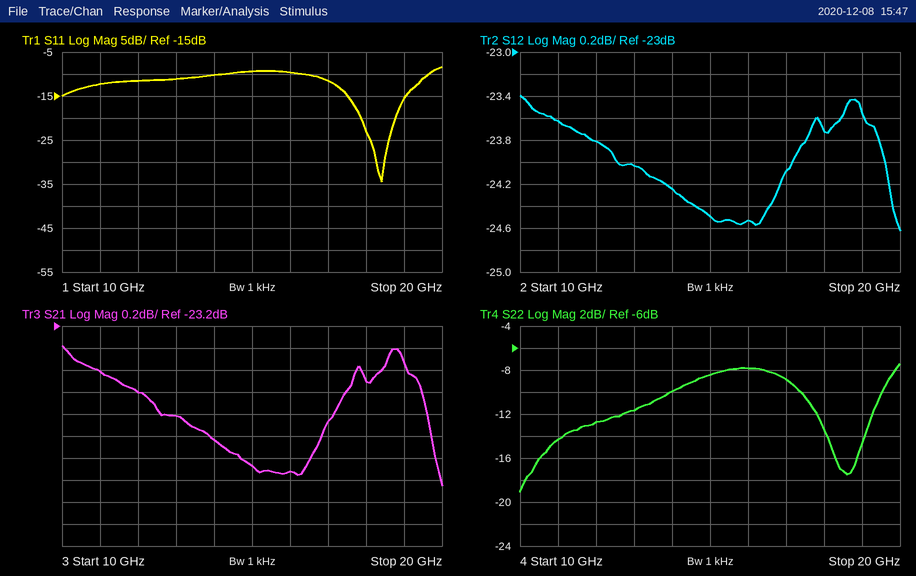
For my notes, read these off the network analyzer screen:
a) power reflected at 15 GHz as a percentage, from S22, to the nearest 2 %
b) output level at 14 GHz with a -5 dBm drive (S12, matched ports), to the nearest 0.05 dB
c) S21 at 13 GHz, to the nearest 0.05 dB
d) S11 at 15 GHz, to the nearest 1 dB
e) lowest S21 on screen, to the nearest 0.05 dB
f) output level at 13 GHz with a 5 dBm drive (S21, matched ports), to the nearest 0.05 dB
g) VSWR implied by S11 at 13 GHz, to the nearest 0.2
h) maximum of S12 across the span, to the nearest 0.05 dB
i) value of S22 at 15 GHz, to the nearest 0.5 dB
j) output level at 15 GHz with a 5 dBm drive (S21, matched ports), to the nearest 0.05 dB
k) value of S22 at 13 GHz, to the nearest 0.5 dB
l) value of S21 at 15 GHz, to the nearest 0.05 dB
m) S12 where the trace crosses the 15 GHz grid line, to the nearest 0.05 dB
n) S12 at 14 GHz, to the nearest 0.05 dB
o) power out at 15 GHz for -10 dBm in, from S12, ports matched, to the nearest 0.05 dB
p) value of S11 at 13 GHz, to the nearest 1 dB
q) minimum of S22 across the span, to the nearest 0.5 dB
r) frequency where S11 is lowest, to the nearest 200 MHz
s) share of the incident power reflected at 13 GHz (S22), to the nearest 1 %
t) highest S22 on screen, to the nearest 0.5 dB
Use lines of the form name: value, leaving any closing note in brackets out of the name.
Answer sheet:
power reflected at 15 GHz as a percentage, from S22, to the nearest 2 %: 14 %
output level at 14 GHz with a -5 dBm drive (S12, matched ports), to the nearest 0.05 dB: -29.25 dBm
S21 at 13 GHz, to the nearest 0.05 dB: -24.00 dB
S11 at 15 GHz, to the nearest 1 dB: -9 dB
lowest S21 on screen, to the nearest 0.05 dB: -24.65 dB
output level at 13 GHz with a 5 dBm drive (S21, matched ports), to the nearest 0.05 dB: -19.00 dBm
VSWR implied by S11 at 13 GHz, to the nearest 0.2: 1.8
maximum of S12 across the span, to the nearest 0.05 dB: -23.40 dB
value of S22 at 15 GHz, to the nearest 0.5 dB: -8.5 dB
output level at 15 GHz with a 5 dBm drive (S21, matched ports), to the nearest 0.05 dB: -19.45 dBm
value of S22 at 13 GHz, to the nearest 0.5 dB: -11.5 dB
value of S21 at 15 GHz, to the nearest 0.05 dB: -24.45 dB
S12 where the trace crosses the 15 GHz grid line, to the nearest 0.05 dB: -24.50 dB
S12 at 14 GHz, to the nearest 0.05 dB: -24.25 dB
power out at 15 GHz for -10 dBm in, from S12, ports matched, to the nearest 0.05 dB: -34.50 dBm
value of S11 at 13 GHz, to the nearest 1 dB: -11 dB
minimum of S22 across the span, to the nearest 0.5 dB: -19.0 dB
frequency where S11 is lowest, to the nearest 200 MHz: 18.4 GHz
share of the incident power reflected at 13 GHz (S22), to the nearest 1 %: 7 %
highest S22 on screen, to the nearest 0.5 dB: -7.5 dB
